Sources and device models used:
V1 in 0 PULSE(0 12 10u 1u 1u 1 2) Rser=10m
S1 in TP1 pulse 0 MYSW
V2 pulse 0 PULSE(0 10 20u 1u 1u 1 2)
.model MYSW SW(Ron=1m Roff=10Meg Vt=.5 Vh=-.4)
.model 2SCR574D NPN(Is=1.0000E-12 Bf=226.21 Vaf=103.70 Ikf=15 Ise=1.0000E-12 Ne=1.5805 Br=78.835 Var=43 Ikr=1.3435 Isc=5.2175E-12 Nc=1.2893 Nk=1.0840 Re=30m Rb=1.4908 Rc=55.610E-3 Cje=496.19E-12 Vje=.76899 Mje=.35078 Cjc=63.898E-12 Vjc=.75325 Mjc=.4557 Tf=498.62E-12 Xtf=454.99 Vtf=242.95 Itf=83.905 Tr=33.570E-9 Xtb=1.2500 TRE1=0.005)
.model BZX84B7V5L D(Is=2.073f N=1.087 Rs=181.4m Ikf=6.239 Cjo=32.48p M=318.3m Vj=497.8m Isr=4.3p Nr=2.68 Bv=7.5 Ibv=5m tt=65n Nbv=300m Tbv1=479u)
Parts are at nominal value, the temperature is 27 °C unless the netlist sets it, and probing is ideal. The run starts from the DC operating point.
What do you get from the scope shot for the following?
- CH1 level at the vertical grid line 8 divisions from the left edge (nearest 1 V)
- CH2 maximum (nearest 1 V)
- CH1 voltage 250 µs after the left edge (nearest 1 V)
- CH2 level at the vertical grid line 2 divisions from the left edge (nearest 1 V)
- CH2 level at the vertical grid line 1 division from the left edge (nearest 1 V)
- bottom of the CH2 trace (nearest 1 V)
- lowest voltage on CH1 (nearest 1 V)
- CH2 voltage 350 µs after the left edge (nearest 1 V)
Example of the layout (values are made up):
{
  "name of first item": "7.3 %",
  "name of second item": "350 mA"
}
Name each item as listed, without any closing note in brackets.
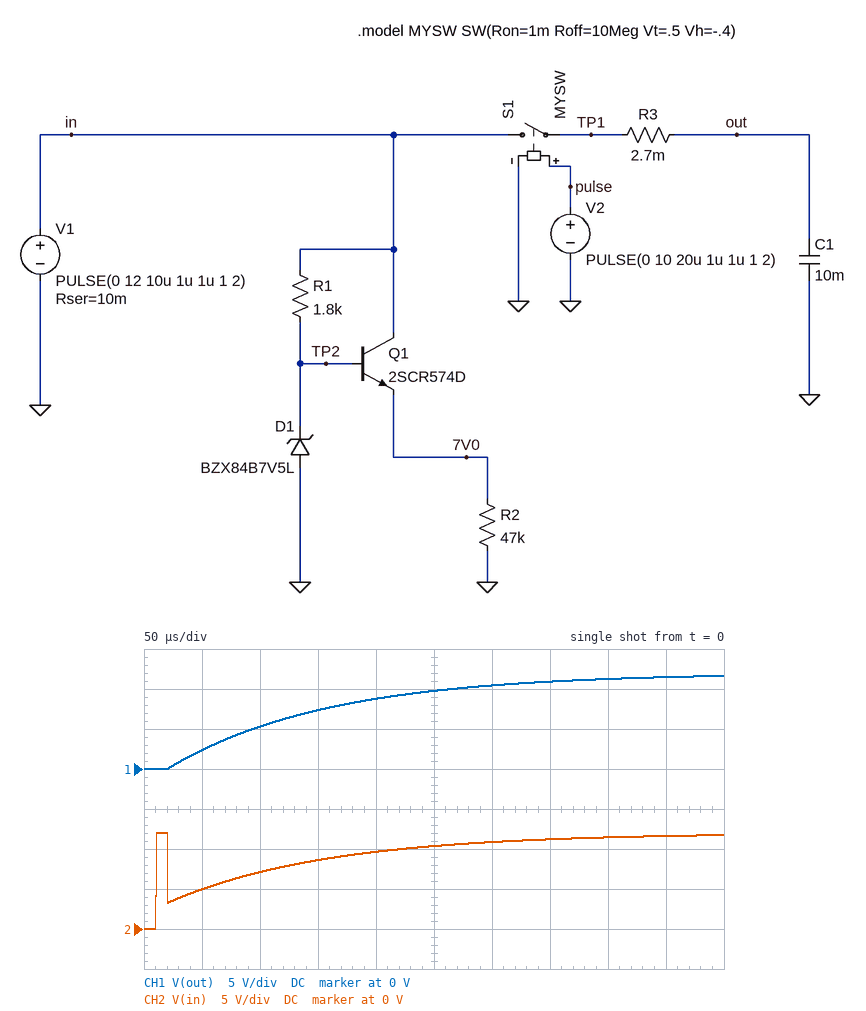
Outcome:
{
  "CH1 level at the vertical grid line 8 divisions from the left edge": "11 V",
  "CH2 maximum": "12 V",
  "CH1 voltage 250 µs after the left edge": "10 V",
  "CH2 level at the vertical grid line 2 divisions from the left edge": "7 V",
  "CH2 level at the vertical grid line 1 division from the left edge": "5 V",
  "bottom of the CH2 trace": "0 V",
  "lowest voltage on CH1": "0 V",
  "CH2 voltage 350 µs after the left edge": "11 V"
}
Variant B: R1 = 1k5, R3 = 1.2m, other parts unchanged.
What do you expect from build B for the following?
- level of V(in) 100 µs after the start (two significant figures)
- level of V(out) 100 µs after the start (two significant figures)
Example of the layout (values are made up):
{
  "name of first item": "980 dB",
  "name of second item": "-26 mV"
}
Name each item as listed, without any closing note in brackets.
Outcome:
{
  "level of V(in) 100 µs after the start": "6.9 V",
  "level of V(out) 100 µs after the start": "5.8 V"
}
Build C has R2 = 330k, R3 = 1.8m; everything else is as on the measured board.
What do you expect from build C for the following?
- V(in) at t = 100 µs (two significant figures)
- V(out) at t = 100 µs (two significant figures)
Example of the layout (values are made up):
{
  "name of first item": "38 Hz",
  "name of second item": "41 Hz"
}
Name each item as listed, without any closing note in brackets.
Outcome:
{
  "V(in) at t = 100 µs": "7.0 V",
  "V(out) at t = 100 µs": "5.6 V"
}
